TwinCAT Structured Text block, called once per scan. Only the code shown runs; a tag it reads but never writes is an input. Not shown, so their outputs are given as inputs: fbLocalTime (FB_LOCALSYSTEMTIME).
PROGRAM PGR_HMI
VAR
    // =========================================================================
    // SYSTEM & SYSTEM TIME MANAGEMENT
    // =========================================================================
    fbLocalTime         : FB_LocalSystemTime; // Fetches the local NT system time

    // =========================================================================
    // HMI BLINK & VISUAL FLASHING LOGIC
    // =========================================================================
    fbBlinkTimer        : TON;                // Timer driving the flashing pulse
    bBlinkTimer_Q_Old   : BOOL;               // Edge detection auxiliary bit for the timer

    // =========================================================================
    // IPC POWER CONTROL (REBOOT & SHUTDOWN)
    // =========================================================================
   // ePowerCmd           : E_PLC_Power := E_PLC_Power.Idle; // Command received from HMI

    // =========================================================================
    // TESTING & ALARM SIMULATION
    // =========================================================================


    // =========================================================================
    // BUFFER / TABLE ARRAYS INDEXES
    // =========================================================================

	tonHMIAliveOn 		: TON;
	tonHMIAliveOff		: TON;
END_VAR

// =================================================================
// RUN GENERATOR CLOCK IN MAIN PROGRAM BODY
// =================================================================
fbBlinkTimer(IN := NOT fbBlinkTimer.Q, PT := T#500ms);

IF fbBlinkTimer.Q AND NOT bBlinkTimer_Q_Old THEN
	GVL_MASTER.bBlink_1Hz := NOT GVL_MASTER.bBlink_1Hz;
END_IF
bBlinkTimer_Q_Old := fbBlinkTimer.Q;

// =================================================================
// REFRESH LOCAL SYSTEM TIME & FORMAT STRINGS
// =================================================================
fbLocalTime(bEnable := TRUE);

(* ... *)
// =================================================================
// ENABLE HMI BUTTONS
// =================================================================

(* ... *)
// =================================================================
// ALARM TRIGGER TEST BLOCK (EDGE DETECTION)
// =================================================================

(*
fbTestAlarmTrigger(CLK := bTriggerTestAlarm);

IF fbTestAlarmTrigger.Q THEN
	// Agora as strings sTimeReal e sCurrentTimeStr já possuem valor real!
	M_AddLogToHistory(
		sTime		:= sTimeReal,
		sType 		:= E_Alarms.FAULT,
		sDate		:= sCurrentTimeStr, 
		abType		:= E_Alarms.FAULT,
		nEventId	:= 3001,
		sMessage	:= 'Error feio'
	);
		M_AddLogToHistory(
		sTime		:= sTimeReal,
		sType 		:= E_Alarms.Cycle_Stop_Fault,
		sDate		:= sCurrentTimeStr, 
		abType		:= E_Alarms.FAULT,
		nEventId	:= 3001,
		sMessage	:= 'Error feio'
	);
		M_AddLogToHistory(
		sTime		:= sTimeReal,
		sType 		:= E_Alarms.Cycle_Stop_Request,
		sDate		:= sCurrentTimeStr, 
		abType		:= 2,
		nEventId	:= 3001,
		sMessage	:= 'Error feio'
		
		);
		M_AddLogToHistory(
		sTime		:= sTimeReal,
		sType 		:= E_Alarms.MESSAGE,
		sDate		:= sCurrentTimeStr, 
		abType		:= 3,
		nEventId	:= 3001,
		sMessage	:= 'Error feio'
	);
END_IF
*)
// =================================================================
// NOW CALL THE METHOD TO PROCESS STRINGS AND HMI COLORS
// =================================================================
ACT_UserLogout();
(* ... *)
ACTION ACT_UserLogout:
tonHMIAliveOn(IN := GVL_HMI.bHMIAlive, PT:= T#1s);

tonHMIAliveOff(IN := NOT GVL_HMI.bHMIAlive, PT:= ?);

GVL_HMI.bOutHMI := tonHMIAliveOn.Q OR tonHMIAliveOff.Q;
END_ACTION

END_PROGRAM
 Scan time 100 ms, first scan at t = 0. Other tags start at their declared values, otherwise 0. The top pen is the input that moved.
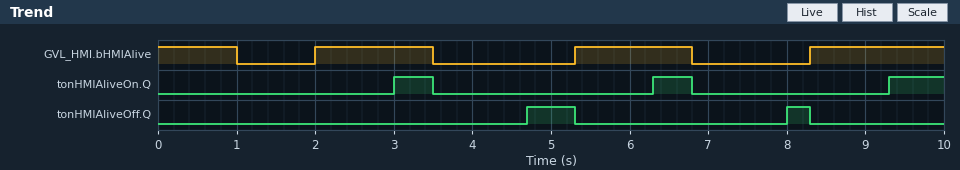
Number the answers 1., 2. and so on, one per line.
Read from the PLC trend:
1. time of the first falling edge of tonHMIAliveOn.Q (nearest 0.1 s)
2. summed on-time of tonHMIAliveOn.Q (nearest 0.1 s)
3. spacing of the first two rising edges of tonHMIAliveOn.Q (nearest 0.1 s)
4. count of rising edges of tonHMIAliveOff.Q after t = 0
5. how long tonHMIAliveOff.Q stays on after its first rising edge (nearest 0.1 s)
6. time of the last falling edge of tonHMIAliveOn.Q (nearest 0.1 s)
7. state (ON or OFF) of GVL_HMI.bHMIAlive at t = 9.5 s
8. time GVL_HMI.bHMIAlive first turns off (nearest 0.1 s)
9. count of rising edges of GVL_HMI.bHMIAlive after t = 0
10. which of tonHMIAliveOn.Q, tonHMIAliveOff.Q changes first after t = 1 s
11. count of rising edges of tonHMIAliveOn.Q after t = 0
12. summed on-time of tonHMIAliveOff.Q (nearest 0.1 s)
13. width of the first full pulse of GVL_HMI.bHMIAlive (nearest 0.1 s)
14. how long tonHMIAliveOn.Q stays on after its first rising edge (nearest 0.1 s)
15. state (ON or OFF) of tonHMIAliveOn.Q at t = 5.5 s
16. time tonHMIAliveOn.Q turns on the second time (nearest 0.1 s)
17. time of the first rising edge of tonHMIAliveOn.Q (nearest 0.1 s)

1. 3.5 s
2. 1.7 s
3. 3.3 s
4. 2
5. 0.6 s
6. 6.8 s
7. ON
8. 1.0 s
9. 3
10. tonHMIAliveOn.Q
11. 3
12. 0.9 s
13. 1.5 s
14. 0.5 s
15. OFF
16. 6.3 s
17. 3.0 s
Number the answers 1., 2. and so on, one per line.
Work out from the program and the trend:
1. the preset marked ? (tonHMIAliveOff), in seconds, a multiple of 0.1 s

1. 1.2 s
